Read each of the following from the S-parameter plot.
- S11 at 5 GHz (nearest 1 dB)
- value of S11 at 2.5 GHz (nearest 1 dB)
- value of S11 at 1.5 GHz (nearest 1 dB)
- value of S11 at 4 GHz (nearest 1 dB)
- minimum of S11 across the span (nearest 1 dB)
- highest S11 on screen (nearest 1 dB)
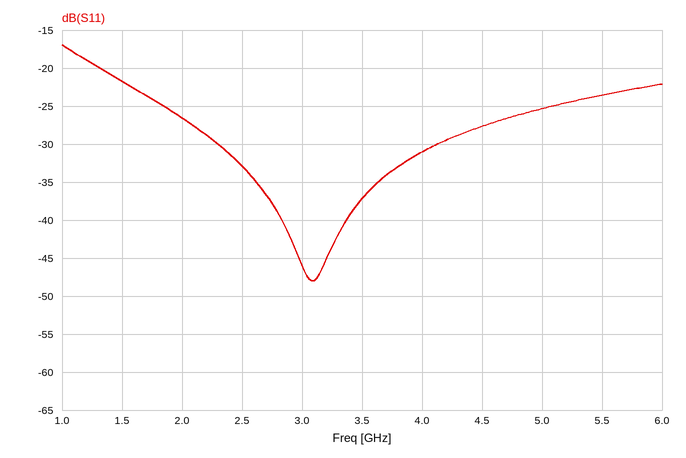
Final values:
-25 dB
-33 dB
-22 dB
-31 dB
-48 dB
-17 dB
